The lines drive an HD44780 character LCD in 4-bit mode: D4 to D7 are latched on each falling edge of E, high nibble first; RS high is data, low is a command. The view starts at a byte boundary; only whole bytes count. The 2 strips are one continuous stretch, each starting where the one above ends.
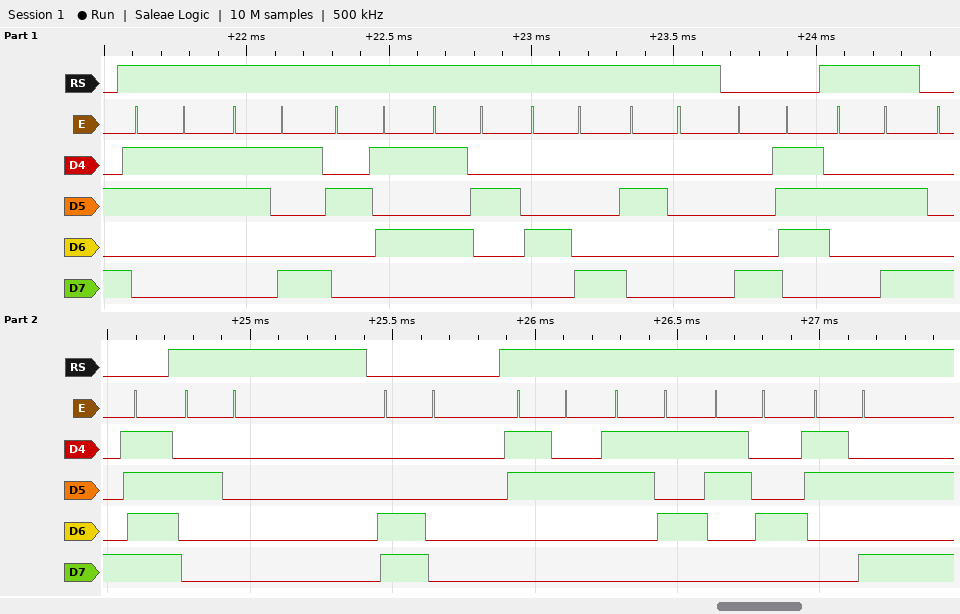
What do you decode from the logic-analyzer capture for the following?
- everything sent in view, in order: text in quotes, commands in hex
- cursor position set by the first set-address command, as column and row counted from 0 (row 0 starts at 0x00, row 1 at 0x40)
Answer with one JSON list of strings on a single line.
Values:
["\"39%RH \" 0x87 \"*\" 0x8F \" \" 0xC0 \"254:\"", "column 7, row 0"]
